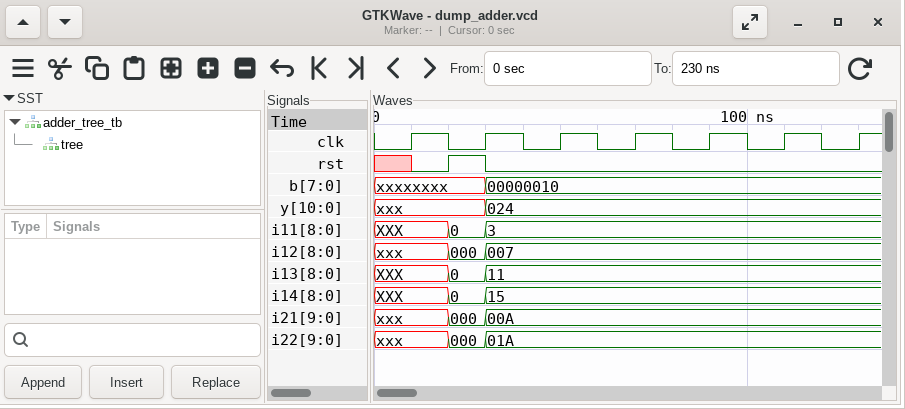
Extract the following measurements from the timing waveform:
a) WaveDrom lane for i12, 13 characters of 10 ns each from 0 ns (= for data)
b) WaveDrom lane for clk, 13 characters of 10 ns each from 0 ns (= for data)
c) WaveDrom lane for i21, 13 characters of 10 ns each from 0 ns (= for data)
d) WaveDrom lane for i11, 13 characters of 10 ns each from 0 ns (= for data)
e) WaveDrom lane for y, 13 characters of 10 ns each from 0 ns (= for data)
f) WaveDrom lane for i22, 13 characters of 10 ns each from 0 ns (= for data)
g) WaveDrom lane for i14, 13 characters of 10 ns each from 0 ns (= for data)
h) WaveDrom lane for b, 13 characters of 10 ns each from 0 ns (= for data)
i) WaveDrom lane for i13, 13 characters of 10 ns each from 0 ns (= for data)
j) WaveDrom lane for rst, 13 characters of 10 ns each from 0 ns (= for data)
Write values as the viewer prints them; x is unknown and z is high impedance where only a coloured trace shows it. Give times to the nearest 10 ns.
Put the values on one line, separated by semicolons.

{name: 'i12', wave: 'x.==.........', data: '000 007'}; {name: 'clk', wave: '0101010101010'}; {name: 'i21', wave: 'x.==.........', data: '000 00A'}; {name: 'i11', wave: 'x.==.........', data: '0 3'}; {name: 'y', wave: 'x..=.........', data: '024'}; {name: 'i22', wave: 'x.==.........', data: '000 01A'}; {name: 'i14', wave: 'x.==.........', data: '0 15'}; {name: 'b', wave: 'x..=.........', data: '00000010'}; {name: 'i13', wave: 'x.==.........', data: '0 11'}; {name: 'rst', wave: 'x010.........'}
